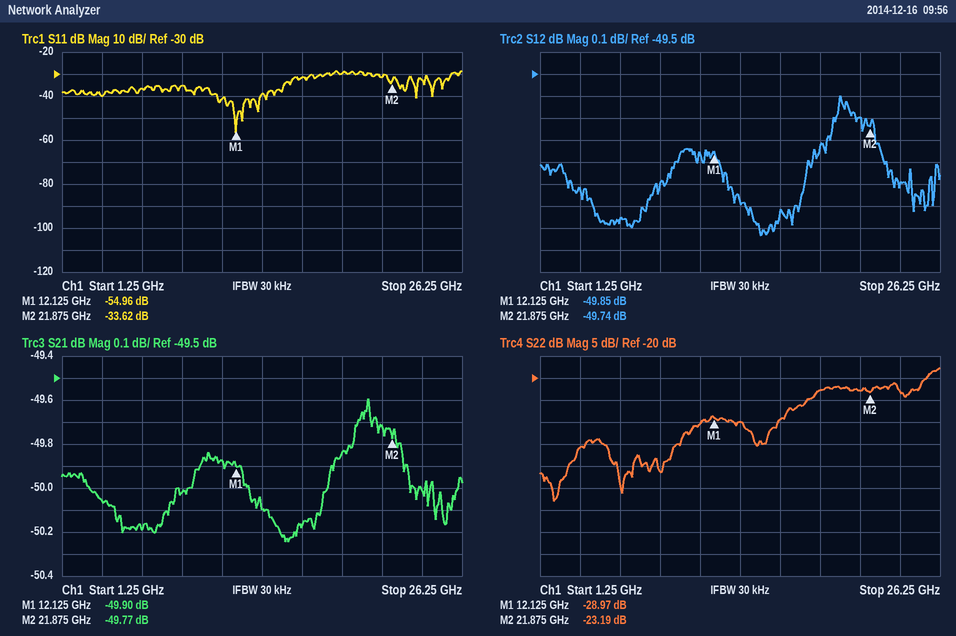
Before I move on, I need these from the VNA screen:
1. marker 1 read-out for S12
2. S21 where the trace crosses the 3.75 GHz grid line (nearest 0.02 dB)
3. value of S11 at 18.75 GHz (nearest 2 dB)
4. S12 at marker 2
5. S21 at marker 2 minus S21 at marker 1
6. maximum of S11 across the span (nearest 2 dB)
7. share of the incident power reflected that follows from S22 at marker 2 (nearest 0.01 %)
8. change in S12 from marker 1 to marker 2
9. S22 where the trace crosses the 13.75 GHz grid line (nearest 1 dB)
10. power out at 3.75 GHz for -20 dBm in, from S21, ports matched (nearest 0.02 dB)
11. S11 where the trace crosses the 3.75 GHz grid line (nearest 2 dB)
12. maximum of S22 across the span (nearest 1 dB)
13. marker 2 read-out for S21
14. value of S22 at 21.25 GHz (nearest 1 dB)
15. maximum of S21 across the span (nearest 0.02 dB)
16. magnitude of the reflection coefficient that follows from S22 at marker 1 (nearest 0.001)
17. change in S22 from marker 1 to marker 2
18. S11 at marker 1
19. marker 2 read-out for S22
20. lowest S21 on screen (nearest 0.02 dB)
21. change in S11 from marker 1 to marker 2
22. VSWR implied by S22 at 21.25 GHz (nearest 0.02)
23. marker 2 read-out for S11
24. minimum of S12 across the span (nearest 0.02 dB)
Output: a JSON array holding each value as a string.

["-49.85 dB", "-50.06 dB", "-30 dB", "-49.74 dB", "0.13 dB", "-28 dB", "0.48 %", "0.11 dB", "-30 dB", "-70.06 dBm", "-40 dB", "-18 dB", "-49.77 dB", "-23 dB", "-49.60 dB", "0.036", "5.78 dB", "-54.96 dB", "-23.19 dB", "-50.24 dB", "21.34 dB", "1.16", "-33.62 dB", "-50.24 dB"]
